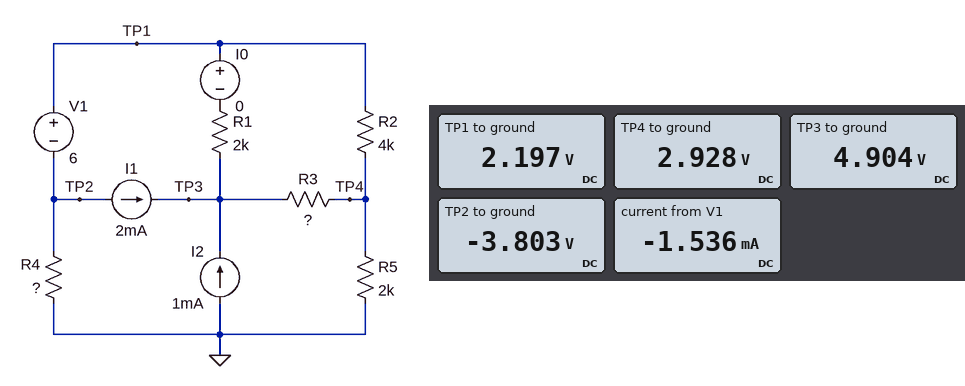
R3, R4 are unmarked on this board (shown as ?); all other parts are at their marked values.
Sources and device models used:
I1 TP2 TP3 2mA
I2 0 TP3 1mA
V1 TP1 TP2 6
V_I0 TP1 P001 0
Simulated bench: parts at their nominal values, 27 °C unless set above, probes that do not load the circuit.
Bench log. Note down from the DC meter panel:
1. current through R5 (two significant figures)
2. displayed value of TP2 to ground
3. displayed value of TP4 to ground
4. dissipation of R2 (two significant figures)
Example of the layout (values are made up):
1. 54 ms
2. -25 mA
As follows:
1. 1.5 mA
2. -3.803 V
3. 2.928 V
4. 130 µW
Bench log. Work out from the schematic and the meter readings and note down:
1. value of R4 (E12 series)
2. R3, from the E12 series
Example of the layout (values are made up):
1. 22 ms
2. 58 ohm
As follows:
1. 8.2 kΩ
2. 1.2 kΩ
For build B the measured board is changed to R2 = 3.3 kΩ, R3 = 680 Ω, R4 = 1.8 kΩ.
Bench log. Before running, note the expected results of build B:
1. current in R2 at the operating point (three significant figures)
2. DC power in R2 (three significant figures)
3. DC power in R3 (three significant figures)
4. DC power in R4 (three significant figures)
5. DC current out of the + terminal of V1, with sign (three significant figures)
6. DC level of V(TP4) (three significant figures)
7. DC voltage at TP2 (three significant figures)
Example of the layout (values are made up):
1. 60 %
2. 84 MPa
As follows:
1. 60.1 µA
2. 11.9 µW
3. 3.19 mW
4. 2.20 mW
5. -895 µA
6. 4.21 V
7. -1.99 V
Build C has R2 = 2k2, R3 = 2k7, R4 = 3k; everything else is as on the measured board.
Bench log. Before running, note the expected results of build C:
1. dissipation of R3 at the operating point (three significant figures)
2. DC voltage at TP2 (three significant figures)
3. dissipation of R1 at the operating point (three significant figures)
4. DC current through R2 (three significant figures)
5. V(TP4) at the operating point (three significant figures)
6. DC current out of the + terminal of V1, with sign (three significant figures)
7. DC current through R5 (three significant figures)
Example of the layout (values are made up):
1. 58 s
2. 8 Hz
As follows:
1. 5.33 mW
2. -2.04 V
3. 5.09 mW
4. 274 µA
5. 3.36 V
6. -1.32 mA
7. 1.68 mA
